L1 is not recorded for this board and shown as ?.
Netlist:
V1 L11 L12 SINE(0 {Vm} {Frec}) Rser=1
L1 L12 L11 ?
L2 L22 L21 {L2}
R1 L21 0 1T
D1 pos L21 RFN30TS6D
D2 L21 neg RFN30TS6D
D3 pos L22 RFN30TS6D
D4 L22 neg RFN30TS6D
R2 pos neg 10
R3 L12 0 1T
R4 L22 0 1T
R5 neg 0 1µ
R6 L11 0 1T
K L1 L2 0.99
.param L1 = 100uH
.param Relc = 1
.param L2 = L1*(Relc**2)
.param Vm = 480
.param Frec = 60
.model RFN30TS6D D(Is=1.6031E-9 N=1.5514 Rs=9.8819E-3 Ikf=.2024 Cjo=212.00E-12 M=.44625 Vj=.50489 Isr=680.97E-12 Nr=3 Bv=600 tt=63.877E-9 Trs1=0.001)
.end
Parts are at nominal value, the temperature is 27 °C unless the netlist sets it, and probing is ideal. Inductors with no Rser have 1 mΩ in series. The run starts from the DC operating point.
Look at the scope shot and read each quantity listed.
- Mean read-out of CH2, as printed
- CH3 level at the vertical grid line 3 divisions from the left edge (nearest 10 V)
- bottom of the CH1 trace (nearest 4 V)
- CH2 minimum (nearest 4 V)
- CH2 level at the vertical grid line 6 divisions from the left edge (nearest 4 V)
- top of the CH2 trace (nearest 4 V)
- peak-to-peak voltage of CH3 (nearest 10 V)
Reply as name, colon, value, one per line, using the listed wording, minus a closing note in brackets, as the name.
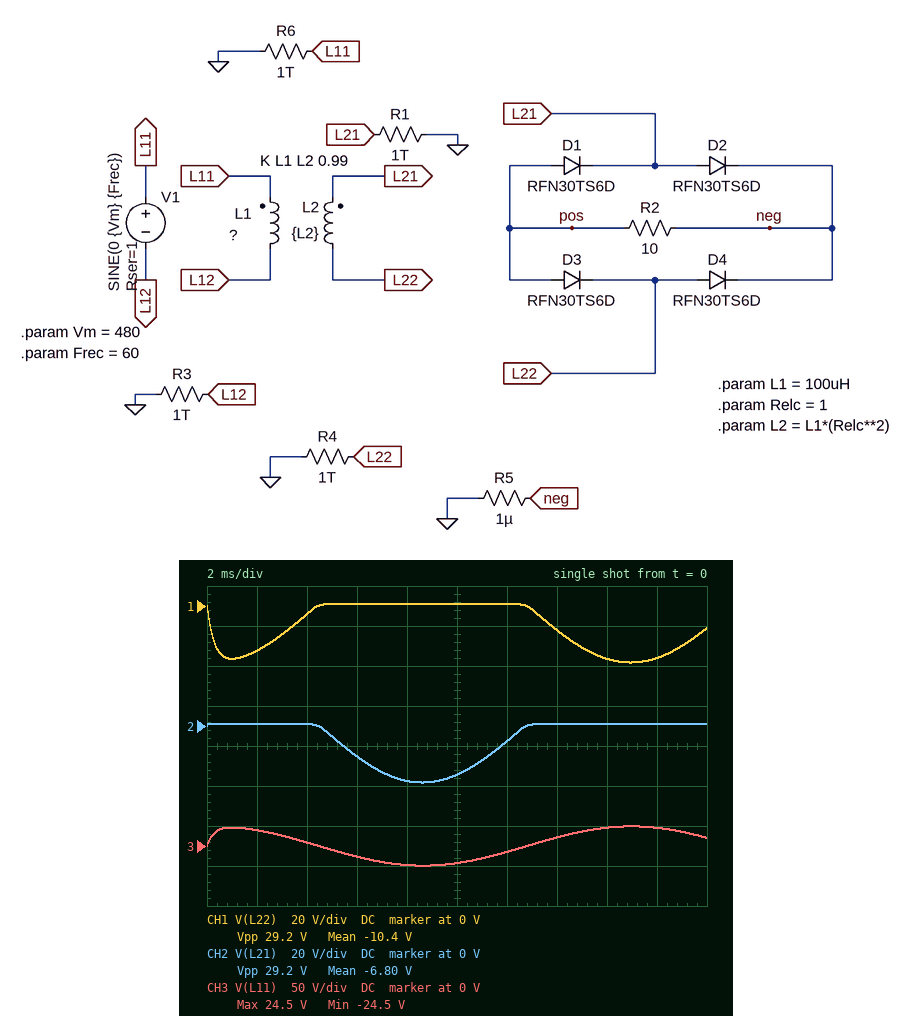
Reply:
Mean read-out of CH2, as printed: -6.80 V
CH3 level at the vertical grid line 3 divisions from the left edge: -10 V
bottom of the CH1 trace: -28 V
CH2 minimum: -28 V
CH2 level at the vertical grid line 6 divisions from the left edge: -8 V
top of the CH2 trace: 0 V
peak-to-peak voltage of CH3: 50 V
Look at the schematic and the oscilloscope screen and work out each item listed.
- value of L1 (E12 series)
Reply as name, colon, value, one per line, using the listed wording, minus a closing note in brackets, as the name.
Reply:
value of L1: 270 µH
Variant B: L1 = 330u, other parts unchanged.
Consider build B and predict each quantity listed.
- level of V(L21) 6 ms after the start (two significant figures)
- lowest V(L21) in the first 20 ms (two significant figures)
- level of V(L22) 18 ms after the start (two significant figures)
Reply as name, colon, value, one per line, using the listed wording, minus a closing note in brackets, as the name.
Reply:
level of V(L21) 6 ms after the start: -16 V
lowest V(L21) in the first 20 ms: -31 V
level of V(L22) 18 ms after the start: -29 V
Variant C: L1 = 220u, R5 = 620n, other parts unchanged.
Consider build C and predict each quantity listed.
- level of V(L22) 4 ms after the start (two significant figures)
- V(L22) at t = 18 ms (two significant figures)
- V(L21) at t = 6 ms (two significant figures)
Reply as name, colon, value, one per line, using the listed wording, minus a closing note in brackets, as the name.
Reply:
level of V(L22) 4 ms after the start: -3.1 V
V(L22) at t = 18 ms: -23 V
V(L21) at t = 6 ms: -14 V
